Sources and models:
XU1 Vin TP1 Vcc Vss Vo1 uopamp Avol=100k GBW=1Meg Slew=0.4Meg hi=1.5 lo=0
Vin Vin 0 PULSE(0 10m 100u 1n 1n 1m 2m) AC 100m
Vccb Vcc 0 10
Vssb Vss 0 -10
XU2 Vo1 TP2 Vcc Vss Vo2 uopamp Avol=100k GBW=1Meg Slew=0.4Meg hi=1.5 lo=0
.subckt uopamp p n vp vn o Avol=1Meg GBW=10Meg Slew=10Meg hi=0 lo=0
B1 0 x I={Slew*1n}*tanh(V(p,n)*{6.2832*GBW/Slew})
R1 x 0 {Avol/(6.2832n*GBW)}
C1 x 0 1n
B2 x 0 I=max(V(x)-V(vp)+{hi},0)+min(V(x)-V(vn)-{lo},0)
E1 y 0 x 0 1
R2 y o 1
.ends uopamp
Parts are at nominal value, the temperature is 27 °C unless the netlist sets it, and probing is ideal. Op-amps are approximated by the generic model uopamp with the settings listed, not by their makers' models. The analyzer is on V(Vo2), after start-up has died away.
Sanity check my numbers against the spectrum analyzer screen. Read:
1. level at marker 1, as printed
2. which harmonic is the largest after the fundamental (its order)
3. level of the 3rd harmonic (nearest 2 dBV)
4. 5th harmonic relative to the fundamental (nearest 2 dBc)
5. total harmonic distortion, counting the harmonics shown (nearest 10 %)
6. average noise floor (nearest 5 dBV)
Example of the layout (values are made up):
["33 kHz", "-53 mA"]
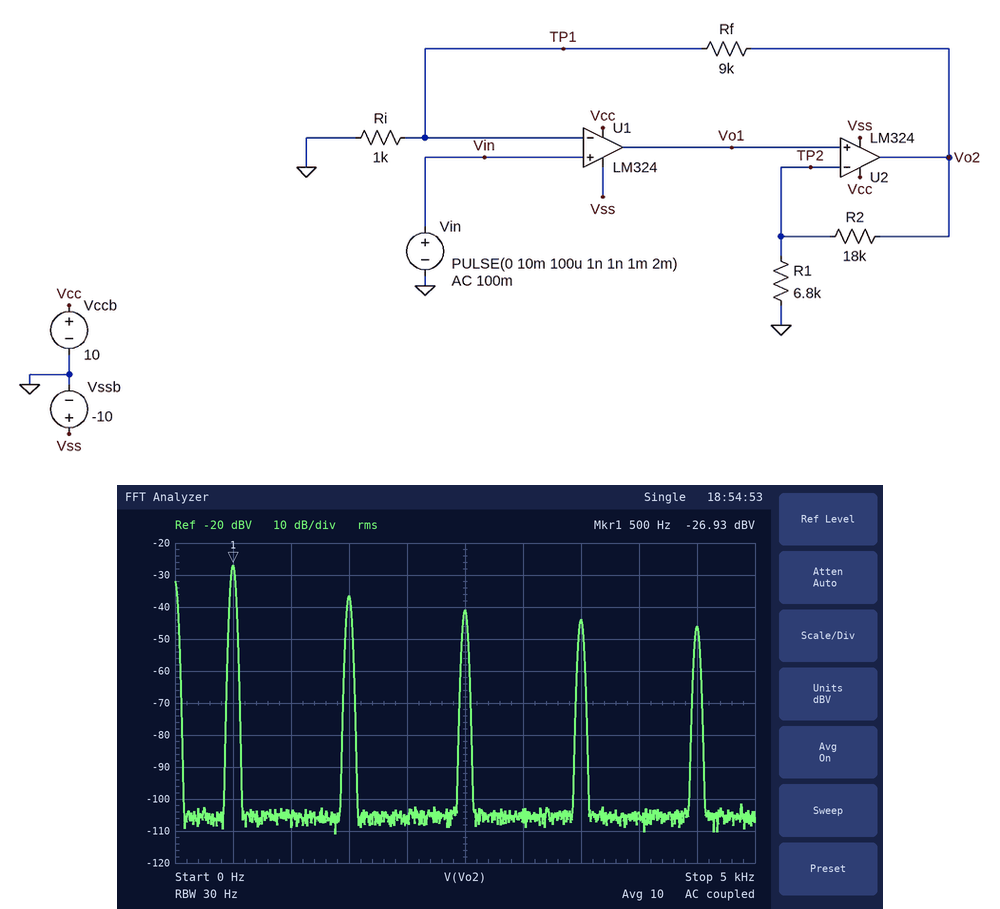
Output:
["-26.93 dBV", "3", "-36 dBV", "-14 dBc", "40 %", "-105 dBV"]
